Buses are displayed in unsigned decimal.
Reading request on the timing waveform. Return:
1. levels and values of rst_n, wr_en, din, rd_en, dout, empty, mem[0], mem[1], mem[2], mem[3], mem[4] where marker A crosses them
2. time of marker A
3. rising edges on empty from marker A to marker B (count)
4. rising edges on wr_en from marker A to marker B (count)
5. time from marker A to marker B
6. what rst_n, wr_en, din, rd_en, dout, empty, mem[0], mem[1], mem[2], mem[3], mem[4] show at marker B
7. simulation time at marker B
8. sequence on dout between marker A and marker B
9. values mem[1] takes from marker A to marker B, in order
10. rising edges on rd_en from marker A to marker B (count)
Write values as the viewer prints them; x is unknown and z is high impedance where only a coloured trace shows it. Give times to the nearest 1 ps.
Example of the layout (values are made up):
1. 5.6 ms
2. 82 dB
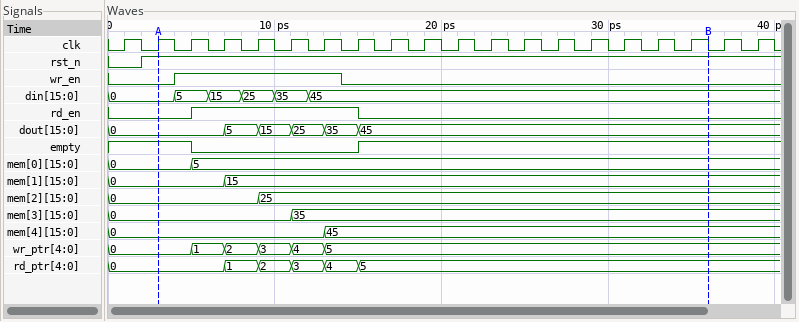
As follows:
1. rst_n=1, wr_en=0, din=0, rd_en=0, dout=0, empty=1, mem[0]=0, mem[1]=0, mem[2]=0, mem[3]=0, mem[4]=0
2. 3 ps
3. 1
4. 1
5. 33 ps
6. rst_n=1, wr_en=0, din=45, rd_en=0, dout=45, empty=1, mem[0]=5, mem[1]=15, mem[2]=25, mem[3]=35, mem[4]=45
7. 36 ps
8. 0, 5, 15, 25, 35, 45
9. 0, 15
10. 1
